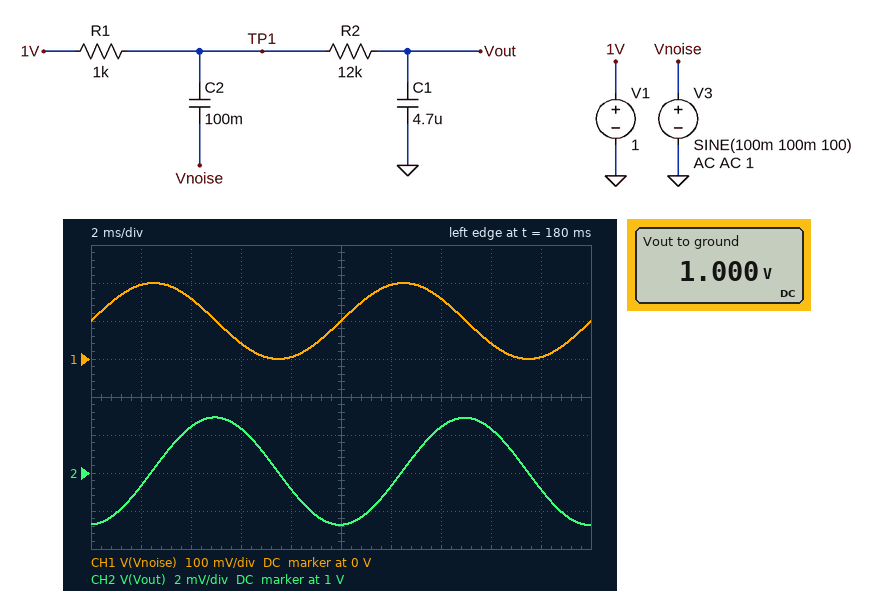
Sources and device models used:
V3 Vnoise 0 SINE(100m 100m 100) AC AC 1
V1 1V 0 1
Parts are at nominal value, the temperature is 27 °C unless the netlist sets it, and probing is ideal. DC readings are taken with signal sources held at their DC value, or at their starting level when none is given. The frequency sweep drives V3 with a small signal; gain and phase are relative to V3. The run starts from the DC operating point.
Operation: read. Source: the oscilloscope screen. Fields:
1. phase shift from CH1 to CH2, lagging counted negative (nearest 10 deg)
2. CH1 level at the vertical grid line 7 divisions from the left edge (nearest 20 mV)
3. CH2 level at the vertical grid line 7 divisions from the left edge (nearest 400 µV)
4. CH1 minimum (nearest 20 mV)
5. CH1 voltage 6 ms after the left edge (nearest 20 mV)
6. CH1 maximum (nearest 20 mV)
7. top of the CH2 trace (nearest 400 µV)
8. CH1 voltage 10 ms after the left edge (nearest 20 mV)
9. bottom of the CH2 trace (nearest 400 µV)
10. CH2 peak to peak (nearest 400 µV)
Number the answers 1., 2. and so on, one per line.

1. -90 deg
2. 160 mV
3. 1.0024 V
4. 0 V
5. 40 mV
6. 200 mV
7. 1.0028 V
8. 100 mV
9. 997.2 mV
10. 5.6 mV
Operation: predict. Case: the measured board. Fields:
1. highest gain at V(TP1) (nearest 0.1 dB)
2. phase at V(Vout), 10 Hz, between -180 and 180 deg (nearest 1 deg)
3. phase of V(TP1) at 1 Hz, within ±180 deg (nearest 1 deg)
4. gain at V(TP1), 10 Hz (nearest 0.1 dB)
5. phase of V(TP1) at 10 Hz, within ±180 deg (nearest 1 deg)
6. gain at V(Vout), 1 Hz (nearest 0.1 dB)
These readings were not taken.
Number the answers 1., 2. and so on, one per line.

1. 0 dB
2. -74 deg
3. 0 deg
4. 0 dB
5. 0 deg
6. -0.5 dB
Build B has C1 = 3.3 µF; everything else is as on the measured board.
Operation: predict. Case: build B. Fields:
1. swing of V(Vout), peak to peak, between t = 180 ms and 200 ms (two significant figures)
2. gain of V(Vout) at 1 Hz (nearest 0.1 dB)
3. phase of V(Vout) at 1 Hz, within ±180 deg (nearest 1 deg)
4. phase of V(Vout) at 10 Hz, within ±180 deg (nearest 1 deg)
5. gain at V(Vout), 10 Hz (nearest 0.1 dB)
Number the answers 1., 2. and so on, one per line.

1. 8.0 mV
2. -0.3 dB
3. -14 deg
4. -68 deg
5. -8.6 dB
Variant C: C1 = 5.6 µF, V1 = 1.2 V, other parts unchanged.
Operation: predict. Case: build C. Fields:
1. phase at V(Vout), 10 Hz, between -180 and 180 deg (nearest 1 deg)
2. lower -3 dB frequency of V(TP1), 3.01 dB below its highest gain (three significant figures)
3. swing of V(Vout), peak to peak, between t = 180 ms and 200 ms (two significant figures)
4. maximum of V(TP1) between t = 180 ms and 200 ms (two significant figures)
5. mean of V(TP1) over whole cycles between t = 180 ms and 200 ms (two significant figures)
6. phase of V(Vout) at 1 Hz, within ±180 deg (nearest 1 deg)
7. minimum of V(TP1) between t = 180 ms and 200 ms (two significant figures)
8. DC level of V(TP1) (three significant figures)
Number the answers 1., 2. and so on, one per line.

1. -77 deg
2. 1.59 mHz
3. 4.8 mV
4. 1.3 V
5. 1.2 V
6. -23 deg
7. 1.1 V
8. 1.20 V
